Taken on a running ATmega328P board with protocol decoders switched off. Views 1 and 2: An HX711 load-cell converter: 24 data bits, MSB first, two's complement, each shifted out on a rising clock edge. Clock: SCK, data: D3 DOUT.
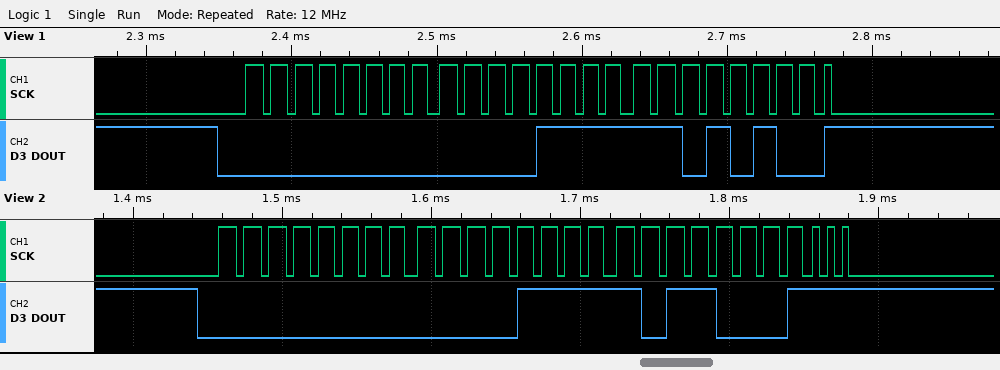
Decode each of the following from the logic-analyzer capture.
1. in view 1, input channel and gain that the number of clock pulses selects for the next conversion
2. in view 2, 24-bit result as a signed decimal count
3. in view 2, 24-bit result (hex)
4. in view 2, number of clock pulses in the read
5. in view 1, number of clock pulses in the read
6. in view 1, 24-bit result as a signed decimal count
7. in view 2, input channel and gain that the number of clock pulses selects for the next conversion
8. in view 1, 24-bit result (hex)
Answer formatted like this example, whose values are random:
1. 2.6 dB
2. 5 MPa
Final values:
1. channel A, gain 128
2. 4017
3. 0x000FB1
4. 27
5. 25
6. 4052
7. channel A, gain 64
8. 0x000FD4
